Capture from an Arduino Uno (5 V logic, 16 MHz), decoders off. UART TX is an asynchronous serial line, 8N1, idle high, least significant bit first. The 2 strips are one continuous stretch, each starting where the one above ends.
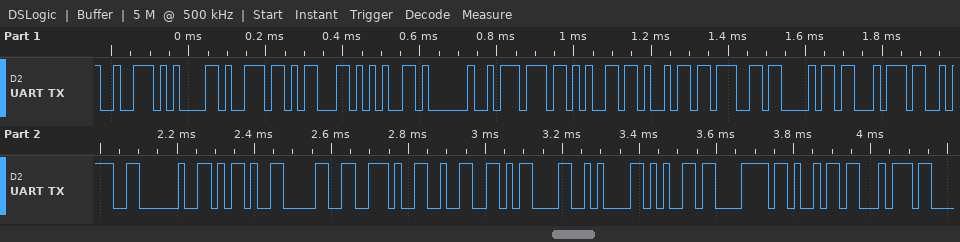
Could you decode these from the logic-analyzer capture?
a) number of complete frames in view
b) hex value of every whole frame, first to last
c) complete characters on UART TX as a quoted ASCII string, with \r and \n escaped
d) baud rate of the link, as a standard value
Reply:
24
72 61 6E 63 65 20 77 65 69 67 68 74 3A 20 2D 30 2E 32 0D 0A 65 78 69 74
"rance weight: -0.2\r\nexit"
57600 baud
